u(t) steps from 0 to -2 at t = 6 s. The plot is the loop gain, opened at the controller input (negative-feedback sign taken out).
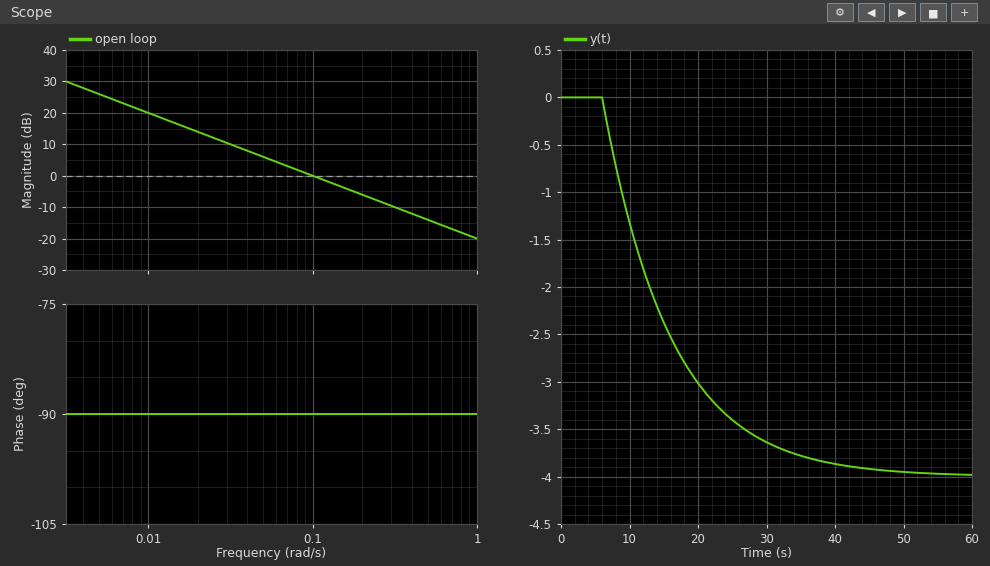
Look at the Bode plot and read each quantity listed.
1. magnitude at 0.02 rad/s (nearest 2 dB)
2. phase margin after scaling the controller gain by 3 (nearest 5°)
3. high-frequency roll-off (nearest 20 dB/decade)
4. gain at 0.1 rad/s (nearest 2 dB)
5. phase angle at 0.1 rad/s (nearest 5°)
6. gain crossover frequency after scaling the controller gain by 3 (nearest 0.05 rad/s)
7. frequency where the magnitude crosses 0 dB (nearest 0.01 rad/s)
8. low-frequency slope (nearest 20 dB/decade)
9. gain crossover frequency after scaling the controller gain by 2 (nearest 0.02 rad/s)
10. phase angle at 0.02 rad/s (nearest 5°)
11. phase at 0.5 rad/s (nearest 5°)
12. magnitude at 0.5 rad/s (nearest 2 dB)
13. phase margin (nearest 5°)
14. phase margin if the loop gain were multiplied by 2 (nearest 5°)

14 dB
90°
-20 dB/decade
0 dB
-90°
0.30 rad/s
0.10 rad/s
-20 dB/decade
0.20 rad/s
-90°
-90°
-14 dB
90°
90°
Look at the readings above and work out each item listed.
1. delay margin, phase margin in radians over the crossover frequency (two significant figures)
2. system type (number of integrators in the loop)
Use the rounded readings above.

16 s
1
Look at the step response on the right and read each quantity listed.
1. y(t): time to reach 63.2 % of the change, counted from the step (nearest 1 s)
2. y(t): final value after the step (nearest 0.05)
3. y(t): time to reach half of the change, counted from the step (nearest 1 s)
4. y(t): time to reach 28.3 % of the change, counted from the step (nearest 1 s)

10 s
-4.00
7 s
3 s
